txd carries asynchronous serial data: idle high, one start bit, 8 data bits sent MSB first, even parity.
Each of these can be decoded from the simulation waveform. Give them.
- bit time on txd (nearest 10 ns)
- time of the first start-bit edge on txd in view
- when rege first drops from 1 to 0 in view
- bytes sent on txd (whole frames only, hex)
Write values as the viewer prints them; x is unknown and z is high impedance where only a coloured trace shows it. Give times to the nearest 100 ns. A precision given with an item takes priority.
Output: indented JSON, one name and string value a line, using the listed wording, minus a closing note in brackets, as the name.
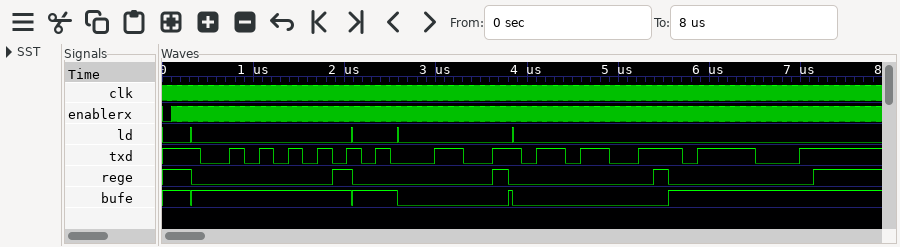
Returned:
{
  "bit time on txd": "160 ns",
  "time of the first start-bit edge on txd in view": "400 ns",
  "when rege first drops from 1 to 0 in view": "300 ns",
  "bytes sent on txd": "55, 8C, D9, F1"
}
